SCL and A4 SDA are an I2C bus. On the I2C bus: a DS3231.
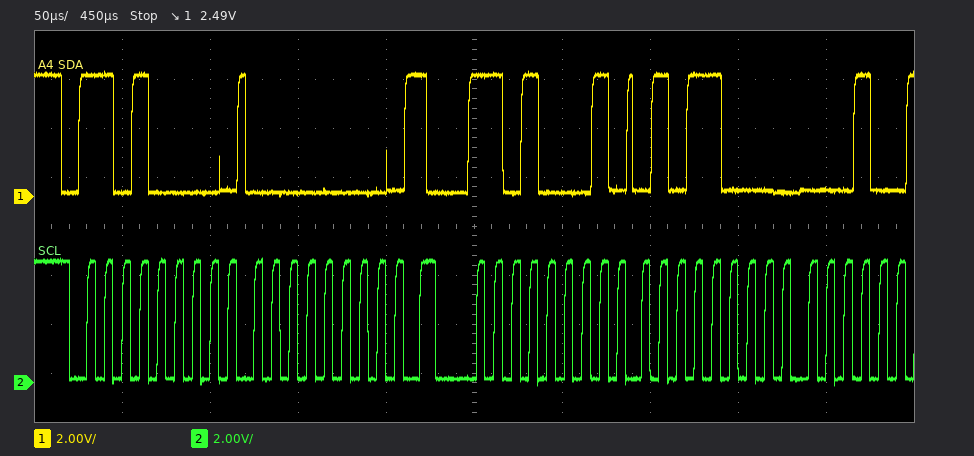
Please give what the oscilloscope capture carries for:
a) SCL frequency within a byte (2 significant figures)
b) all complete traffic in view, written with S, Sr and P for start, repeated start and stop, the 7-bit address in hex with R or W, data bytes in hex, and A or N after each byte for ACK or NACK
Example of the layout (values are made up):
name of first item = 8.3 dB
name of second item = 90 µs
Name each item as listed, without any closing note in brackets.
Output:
SCL frequency within a byte = 100 kHz
all complete traffic in view, written with S, Sr and P for start, repeated start and stop, the 7-bit address in hex with R or W, data bytes in hex, and A or N after each byte for ACK or NACK = S 68W A 00 A Sr 68R A 58 A
